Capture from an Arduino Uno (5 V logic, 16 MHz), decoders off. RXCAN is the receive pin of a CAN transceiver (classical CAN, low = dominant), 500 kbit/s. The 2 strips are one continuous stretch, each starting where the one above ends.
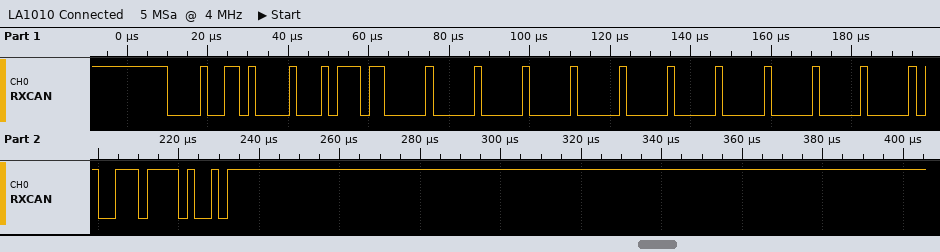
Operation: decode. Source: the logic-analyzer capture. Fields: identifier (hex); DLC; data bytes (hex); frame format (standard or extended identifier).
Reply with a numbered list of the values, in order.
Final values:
1. 0x09A
2. 8
3. BB 00 00 00 00 00 00 00
4. standard
